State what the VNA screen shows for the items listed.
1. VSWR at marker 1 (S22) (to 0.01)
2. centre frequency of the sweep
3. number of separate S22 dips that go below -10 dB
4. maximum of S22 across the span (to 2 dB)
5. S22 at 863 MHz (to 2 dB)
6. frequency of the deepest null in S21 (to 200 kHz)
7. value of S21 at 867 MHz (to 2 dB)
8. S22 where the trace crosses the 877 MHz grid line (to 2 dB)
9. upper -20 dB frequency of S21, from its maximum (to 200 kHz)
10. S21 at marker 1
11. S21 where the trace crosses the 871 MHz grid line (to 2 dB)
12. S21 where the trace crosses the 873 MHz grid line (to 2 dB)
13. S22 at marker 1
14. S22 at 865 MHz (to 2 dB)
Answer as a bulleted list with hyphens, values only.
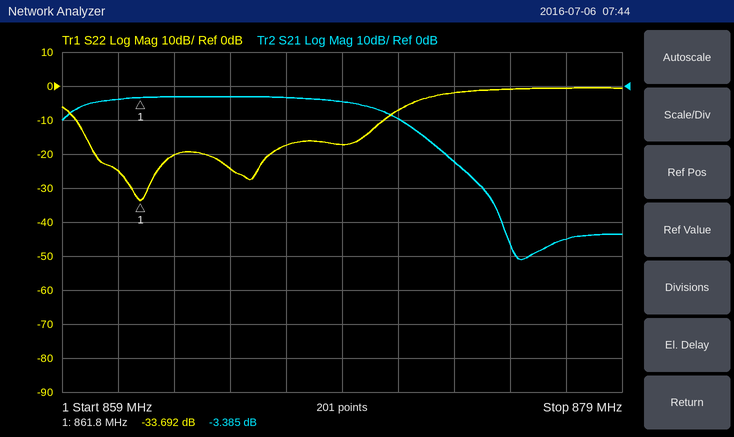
- 1.04
- 869 MHz
- 2
- 0 dB
- -20 dB
- 875.4 MHz
- -4 dB
- 0 dB
- 873.2 MHz
- -3.385 dB
- -10 dB
- -22 dB
- -33.692 dB
- -24 dB
